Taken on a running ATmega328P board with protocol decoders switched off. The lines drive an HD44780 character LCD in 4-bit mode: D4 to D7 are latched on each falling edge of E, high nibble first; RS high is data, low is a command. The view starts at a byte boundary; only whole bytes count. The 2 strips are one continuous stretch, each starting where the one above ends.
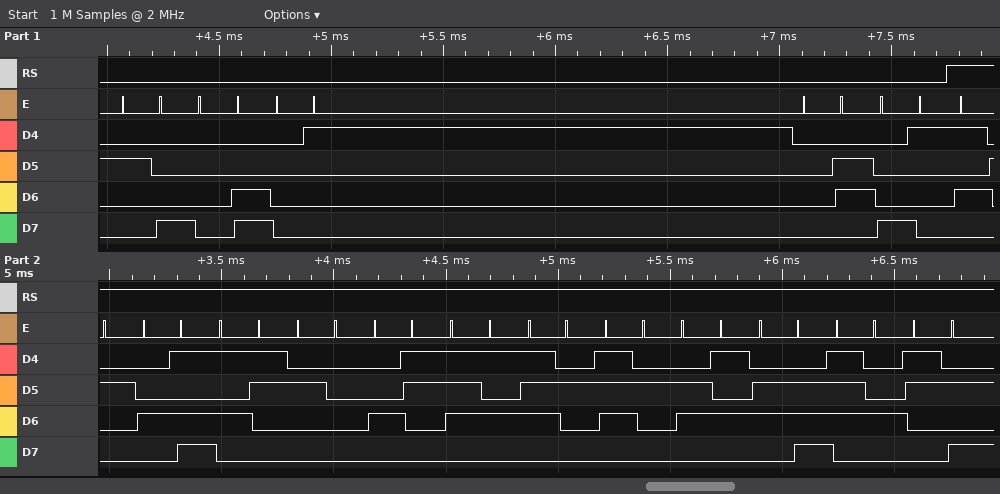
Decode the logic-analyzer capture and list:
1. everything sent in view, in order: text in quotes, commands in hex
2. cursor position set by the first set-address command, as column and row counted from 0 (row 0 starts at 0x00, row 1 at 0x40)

0x28 0x0C 0x01 0x06 0x81 "RMS Current:"
column 1, row 0
